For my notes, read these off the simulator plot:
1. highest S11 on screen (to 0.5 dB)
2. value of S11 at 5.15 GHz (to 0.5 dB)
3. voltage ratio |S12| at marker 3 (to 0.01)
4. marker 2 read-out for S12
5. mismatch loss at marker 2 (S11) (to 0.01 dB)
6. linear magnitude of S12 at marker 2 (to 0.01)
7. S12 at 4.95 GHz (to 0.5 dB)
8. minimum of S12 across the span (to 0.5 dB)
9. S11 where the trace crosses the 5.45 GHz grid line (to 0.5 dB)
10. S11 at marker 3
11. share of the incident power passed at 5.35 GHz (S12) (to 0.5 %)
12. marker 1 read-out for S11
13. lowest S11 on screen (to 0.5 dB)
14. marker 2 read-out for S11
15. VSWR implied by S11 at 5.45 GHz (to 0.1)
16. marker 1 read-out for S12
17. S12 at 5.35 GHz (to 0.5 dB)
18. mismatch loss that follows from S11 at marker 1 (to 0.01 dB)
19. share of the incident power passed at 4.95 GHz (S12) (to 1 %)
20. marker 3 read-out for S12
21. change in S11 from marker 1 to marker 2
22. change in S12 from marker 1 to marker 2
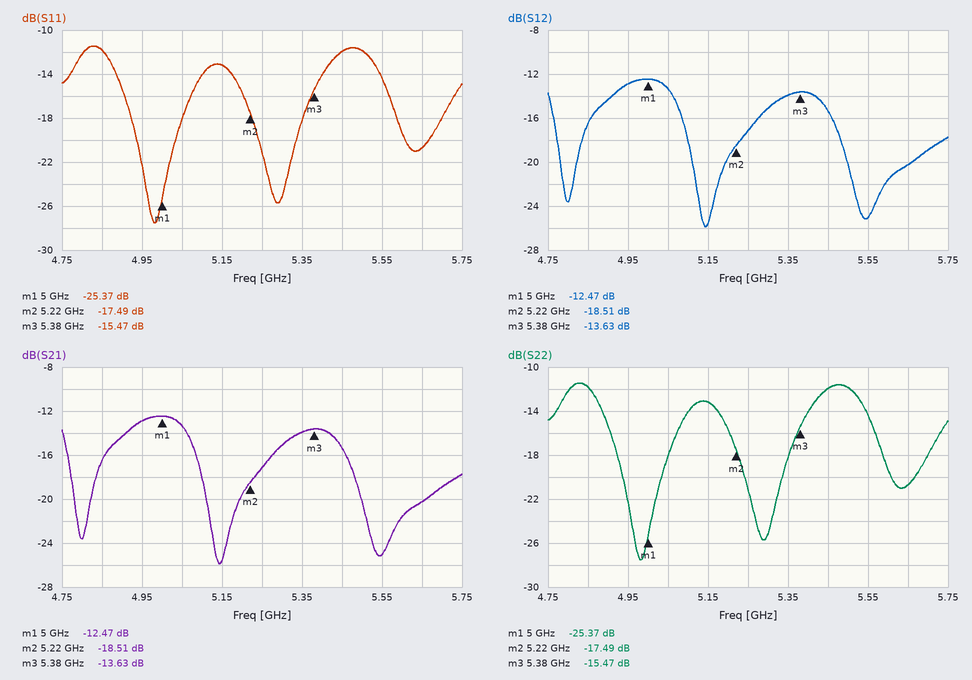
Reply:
-11.5 dB
-13.0 dB
0.21
-18.51 dB
0.08 dB
0.12
-13.0 dB
-26.0 dB
-12.0 dB
-15.47 dB
4.0 %
-25.37 dB
-27.5 dB
-17.49 dB
1.7
-12.47 dB
-14.0 dB
0.01 dB
5 %
-13.63 dB
7.88 dB
-6.04 dB
